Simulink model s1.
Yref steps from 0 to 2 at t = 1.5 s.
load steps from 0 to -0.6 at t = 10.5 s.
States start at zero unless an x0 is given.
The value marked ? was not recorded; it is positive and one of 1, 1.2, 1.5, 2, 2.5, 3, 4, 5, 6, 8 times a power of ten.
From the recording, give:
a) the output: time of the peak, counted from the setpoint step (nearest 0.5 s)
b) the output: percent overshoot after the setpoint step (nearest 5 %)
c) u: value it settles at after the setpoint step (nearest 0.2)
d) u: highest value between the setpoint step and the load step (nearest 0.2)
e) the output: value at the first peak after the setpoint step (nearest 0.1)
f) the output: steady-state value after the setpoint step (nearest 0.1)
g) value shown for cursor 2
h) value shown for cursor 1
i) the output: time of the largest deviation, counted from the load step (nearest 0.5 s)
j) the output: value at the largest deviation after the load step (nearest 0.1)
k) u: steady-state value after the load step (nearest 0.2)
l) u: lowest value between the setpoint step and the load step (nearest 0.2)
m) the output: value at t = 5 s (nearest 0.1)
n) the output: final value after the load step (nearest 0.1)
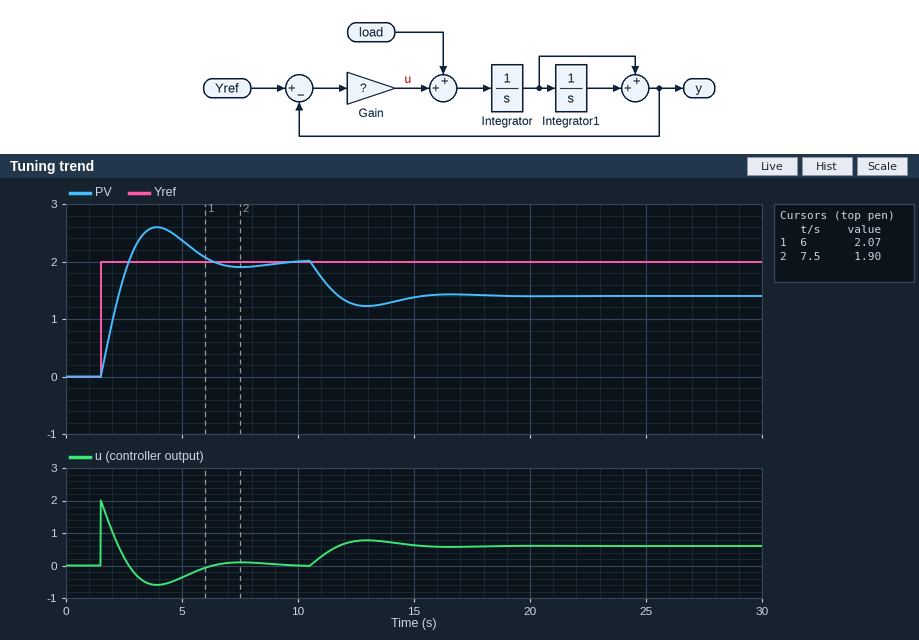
2.5 s
30 %
0.0
2.0
2.6
2.0
1.90
2.07
2.5 s
1.2
0.6
-0.6
2.4
1.4
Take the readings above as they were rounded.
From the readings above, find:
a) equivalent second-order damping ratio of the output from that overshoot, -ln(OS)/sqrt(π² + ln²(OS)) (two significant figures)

0.36
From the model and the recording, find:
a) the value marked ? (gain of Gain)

1
